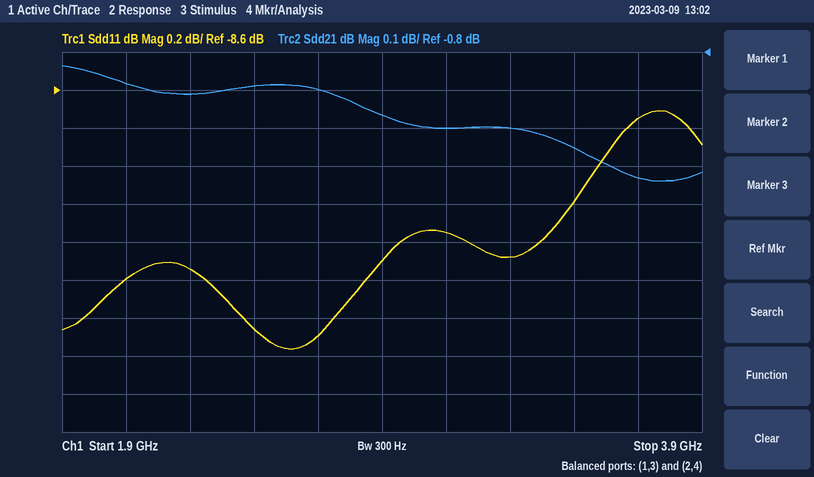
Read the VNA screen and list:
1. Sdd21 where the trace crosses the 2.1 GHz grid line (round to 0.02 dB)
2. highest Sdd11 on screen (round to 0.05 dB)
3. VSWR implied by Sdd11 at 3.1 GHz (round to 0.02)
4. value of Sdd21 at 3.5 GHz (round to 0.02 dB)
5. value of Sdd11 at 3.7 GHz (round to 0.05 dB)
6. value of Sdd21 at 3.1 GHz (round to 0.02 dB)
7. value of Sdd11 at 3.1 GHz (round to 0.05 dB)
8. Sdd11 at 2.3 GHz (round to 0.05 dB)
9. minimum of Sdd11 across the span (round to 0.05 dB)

-0.88 dB
-8.70 dB
2.04
-1.06 dB
-8.75 dB
-1.00 dB
-9.35 dB
-9.55 dB
-9.95 dB
